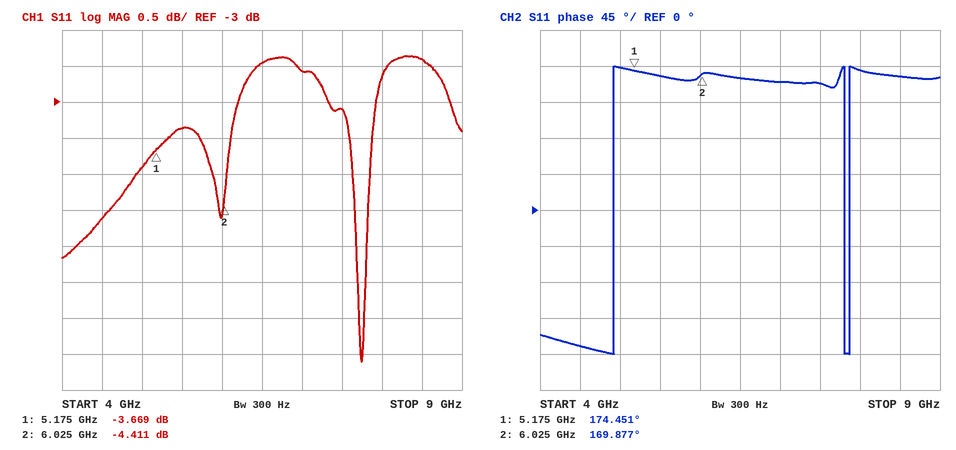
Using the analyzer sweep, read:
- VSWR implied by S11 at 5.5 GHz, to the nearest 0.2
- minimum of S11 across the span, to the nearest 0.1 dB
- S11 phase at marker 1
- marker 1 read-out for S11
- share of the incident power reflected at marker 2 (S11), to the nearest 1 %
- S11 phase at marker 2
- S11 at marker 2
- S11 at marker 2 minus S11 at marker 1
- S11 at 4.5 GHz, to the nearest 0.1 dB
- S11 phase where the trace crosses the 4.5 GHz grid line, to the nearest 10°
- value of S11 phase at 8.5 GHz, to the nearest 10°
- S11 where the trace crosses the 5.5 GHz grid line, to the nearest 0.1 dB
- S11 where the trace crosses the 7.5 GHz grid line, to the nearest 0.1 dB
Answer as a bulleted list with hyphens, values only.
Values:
- 5.2
- -6.6 dB
- 174.451°
- -3.669 dB
- 36 %
- 169.877°
- -4.411 dB
- -0.742 dB
- -4.6 dB
- -170°
- 170°
- -3.4 dB
- -3.1 dB
